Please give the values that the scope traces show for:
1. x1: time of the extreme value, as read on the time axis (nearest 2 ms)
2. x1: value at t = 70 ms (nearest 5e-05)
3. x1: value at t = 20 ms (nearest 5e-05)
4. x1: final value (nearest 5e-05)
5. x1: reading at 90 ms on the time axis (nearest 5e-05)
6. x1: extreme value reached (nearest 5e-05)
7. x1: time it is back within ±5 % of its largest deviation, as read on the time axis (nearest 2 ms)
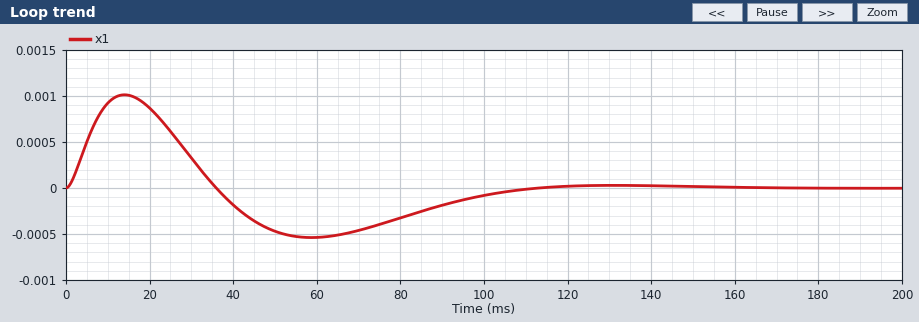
14 ms
-0.00045
0.00085
0.00000
-0.00020
0.00100
104 ms
